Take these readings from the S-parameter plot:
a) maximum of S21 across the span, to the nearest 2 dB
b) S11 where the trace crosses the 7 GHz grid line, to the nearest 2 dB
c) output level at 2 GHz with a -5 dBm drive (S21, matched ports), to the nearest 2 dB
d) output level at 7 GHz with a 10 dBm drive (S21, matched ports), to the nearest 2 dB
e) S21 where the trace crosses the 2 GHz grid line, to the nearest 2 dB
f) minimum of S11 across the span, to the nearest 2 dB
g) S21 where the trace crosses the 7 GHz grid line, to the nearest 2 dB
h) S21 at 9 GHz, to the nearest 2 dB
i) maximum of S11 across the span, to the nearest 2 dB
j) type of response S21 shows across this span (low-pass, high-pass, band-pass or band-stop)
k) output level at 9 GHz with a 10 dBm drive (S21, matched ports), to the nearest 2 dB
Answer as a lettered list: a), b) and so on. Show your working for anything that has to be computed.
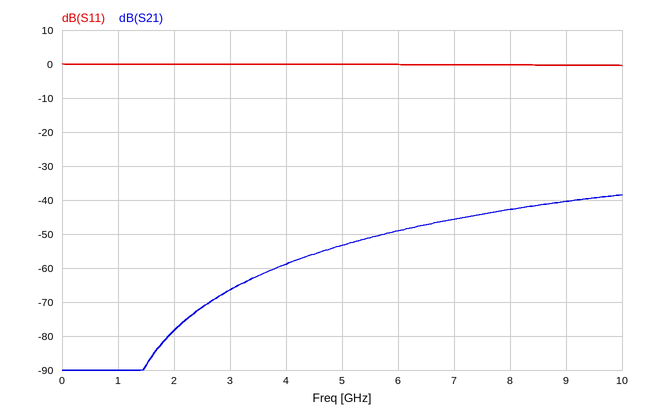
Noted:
a) -38 dB
b) 0 dB
c) -5 dBm + (-78 dB) = -84 dBm
d) 10 dBm + (-46 dB) = -36 dBm
e) -78 dB
f) 0 dB
g) -46 dB
h) -40 dB
i) 0 dB
j) high-pass
k) 10 dBm + (-40 dB) = -30 dBm
